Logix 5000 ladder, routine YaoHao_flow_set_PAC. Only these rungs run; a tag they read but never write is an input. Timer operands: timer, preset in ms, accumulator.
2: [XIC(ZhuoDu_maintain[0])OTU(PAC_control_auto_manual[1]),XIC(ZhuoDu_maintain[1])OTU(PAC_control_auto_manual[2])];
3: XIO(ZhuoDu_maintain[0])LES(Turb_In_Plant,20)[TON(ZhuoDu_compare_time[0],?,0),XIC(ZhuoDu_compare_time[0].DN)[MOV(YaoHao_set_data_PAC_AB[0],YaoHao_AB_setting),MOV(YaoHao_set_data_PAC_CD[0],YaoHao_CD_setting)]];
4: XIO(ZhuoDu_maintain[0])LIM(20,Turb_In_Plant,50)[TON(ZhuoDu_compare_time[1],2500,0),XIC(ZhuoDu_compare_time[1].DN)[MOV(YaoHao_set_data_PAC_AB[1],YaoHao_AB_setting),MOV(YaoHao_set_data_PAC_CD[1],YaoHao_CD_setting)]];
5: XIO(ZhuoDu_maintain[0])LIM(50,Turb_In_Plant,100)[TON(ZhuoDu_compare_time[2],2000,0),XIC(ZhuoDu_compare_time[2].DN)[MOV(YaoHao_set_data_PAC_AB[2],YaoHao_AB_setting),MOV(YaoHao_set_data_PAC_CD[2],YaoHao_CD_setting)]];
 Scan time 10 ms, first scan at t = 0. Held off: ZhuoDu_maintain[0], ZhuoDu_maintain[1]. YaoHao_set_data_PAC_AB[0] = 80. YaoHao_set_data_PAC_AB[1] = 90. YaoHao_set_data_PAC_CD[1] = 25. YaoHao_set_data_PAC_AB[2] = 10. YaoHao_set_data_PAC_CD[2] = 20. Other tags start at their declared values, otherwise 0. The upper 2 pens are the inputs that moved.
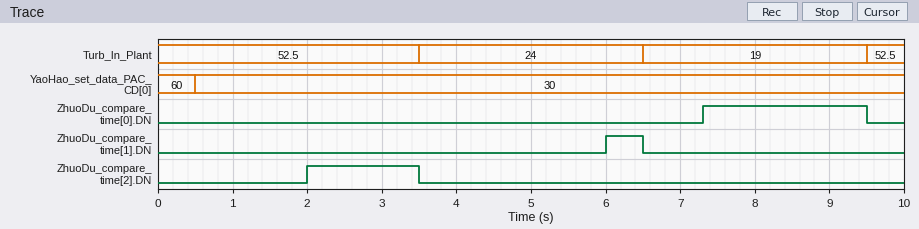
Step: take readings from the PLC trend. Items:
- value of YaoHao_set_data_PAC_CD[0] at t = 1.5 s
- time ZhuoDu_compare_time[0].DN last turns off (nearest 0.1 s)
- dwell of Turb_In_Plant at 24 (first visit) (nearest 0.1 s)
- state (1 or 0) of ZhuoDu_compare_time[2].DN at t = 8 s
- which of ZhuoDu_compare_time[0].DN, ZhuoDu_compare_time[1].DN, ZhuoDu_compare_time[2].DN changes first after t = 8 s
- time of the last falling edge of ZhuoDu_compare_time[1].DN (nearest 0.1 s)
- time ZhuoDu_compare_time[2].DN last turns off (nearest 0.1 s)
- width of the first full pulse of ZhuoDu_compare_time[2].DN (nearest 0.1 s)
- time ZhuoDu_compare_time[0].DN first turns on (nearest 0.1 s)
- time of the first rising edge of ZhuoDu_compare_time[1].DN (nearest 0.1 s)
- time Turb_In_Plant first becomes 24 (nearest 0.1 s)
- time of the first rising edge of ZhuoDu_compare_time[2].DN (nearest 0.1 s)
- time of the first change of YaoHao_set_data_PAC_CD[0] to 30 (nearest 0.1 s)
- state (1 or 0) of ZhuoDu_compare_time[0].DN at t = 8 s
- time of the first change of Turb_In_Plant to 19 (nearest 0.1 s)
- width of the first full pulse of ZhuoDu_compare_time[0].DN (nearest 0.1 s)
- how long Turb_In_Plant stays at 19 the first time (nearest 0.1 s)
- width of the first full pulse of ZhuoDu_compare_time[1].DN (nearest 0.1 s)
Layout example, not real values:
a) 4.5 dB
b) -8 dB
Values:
a) 30
b) 9.5 s
c) 3.0 s
d) 0
e) ZhuoDu_compare_time[0].DN
f) 6.5 s
g) 3.5 s
h) 1.5 s
i) 7.3 s
j) 6.0 s
k) 3.5 s
l) 2.0 s
m) 0.5 s
n) 1
o) 6.5 s
p) 2.2 s
q) 3.0 s
r) 0.5 s
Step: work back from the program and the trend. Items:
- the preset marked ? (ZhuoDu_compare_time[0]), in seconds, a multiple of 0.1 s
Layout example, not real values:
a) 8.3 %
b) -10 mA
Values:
a) 0.8 s
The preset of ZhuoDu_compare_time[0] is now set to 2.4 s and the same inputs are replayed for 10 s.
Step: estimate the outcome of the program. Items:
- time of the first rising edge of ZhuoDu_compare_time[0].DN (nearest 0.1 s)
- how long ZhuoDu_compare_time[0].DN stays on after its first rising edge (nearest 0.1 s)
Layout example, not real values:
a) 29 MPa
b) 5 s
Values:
a) 8.9 s
b) 0.6 s
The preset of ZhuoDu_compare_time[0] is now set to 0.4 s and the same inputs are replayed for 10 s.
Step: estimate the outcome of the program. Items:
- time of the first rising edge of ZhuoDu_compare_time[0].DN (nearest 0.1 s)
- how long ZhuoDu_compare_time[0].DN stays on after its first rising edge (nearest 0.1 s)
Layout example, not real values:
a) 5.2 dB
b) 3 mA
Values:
a) 6.9 s
b) 2.6 s
